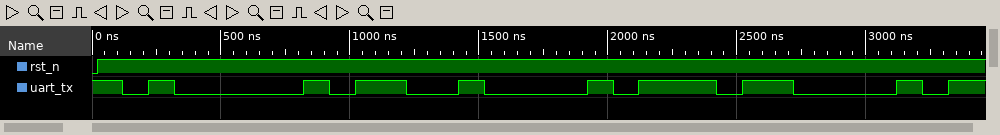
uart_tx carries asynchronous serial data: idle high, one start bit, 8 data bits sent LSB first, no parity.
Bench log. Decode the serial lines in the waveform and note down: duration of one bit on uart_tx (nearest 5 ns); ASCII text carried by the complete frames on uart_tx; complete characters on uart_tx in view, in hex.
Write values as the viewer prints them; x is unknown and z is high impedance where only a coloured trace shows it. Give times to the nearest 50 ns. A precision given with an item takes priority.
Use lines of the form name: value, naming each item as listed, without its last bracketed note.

duration of one bit on uart_tx: 100 ns
ASCII text carried by the complete frames on uart_tx: "ABC"
complete characters on uart_tx in view, in hex: 41, 42, 43
